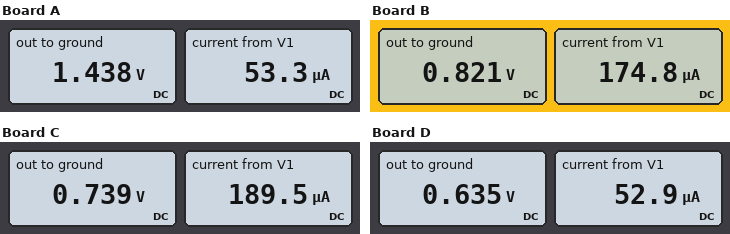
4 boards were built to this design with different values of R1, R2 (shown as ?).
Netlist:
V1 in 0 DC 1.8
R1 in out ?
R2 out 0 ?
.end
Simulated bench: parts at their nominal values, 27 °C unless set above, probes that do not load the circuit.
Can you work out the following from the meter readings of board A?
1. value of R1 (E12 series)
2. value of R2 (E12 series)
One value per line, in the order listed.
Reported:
6.8 kΩ
27 kΩ
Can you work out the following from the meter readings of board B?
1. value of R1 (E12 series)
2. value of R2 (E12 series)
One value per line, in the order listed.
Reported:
5.6 kΩ
4.7 kΩ
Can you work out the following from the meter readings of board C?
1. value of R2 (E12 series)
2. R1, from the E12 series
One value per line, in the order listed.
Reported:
3.9 kΩ
5.6 kΩ
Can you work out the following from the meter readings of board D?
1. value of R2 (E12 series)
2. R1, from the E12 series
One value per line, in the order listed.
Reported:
12 kΩ
22 kΩ
